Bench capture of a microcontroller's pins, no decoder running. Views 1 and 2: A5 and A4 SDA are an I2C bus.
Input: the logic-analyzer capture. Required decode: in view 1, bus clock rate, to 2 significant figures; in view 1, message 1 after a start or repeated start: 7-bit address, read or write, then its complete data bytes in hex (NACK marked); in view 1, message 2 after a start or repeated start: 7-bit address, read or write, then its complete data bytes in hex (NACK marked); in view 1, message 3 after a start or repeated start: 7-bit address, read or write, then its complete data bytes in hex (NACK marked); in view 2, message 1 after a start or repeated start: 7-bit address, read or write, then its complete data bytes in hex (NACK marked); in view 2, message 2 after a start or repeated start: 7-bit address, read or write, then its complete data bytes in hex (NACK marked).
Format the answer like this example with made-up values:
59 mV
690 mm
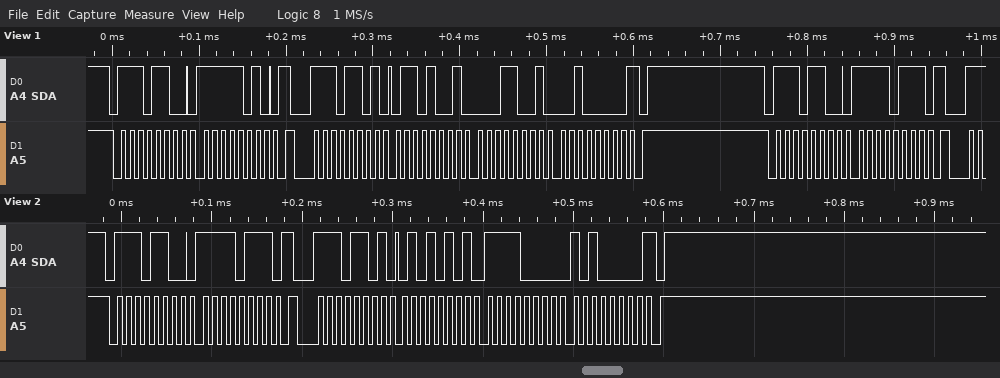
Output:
100 kHz
0x76 write: FA
0x76 read: 69 19 20 NACK
0x76 write: F7
0x76 write: F7
0x76 read: 55 F0 A0 NACK
